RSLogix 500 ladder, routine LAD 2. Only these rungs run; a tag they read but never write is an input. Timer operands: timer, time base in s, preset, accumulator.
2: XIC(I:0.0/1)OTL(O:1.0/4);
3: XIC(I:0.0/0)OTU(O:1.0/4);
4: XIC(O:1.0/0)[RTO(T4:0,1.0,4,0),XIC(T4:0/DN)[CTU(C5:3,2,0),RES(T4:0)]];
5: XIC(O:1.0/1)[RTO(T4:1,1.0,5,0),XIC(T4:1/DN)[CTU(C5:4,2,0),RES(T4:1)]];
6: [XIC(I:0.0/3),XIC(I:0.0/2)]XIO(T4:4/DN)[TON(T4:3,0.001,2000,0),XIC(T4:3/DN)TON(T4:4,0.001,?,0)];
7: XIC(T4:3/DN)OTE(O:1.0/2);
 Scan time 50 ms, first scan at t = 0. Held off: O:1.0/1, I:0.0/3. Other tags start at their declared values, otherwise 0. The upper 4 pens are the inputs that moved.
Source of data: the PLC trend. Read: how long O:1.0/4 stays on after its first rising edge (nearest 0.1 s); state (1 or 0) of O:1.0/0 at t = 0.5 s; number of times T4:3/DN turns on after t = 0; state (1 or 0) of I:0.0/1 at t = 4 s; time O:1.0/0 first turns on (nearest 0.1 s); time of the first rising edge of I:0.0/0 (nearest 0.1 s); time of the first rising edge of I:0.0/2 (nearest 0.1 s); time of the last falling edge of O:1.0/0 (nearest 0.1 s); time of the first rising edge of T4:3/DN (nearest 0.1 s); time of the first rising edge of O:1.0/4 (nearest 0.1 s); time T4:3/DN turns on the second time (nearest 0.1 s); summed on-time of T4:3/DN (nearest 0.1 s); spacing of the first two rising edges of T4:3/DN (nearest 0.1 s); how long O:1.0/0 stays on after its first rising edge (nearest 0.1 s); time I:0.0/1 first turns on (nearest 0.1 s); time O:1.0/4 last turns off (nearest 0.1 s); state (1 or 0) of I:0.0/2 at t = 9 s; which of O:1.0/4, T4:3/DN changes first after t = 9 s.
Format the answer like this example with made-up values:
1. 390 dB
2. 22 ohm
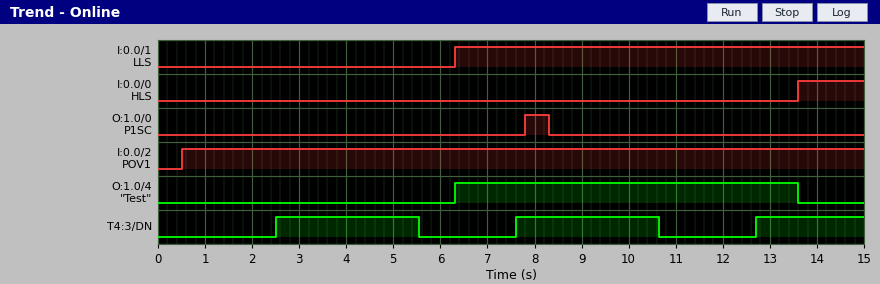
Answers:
1. 7.3 s
2. 0
3. 3
4. 0
5. 7.8 s
6. 13.6 s
7. 0.5 s
8. 8.3 s
9. 2.5 s
10. 6.3 s
11. 7.6 s
12. 8.4 s
13. 5.1 s
14. 0.5 s
15. 6.3 s
16. 13.6 s
17. 1
18. T4:3/DN
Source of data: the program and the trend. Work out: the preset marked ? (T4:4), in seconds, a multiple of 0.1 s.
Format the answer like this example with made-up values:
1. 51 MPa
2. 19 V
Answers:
1. 3.0 s
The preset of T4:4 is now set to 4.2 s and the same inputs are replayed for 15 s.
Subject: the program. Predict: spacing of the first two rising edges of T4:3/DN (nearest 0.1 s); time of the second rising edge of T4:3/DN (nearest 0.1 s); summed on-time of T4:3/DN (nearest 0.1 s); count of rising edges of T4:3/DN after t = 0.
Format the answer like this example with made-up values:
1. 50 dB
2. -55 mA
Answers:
1. 6.3 s
2. 8.8 s
3. 8.5 s
4. 2
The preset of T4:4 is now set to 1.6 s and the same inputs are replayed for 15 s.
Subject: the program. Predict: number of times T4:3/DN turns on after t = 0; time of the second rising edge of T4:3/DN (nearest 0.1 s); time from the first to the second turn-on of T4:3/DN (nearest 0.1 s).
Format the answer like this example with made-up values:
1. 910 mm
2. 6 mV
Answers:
1. 4
2. 6.2 s
3. 3.7 s
